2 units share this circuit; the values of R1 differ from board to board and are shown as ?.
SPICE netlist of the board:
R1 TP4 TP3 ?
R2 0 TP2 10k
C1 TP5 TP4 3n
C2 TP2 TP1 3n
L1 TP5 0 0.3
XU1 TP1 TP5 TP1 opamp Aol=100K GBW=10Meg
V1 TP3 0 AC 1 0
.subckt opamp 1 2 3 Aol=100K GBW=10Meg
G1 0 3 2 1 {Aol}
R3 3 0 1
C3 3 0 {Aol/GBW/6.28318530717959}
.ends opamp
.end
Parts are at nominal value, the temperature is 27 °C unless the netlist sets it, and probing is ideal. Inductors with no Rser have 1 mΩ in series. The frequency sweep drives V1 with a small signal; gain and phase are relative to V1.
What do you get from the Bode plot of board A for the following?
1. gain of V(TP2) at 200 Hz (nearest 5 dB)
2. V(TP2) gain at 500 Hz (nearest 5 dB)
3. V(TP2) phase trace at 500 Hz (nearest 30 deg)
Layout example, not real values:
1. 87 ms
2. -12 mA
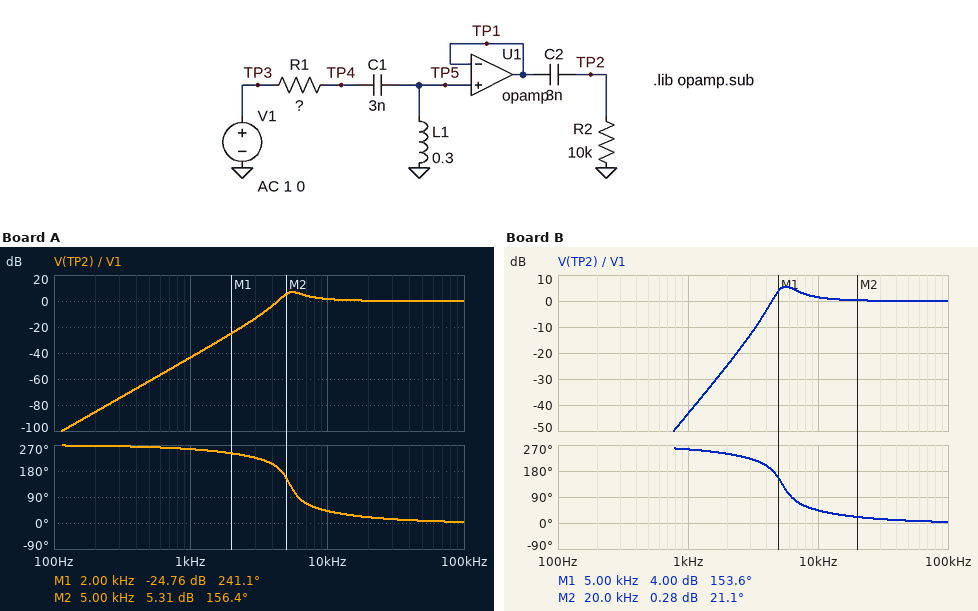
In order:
1. -85 dB
2. -60 dB
3. 270 deg
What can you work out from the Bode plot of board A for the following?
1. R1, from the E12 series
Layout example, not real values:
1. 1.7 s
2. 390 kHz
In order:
1. 3.3 kΩ
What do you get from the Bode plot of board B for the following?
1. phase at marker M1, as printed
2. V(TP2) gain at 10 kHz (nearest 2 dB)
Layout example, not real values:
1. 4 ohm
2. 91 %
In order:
1. 153.6 deg
2. 2 dB
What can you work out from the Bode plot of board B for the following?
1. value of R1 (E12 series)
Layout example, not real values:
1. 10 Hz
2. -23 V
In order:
1. 3.9 kΩ
